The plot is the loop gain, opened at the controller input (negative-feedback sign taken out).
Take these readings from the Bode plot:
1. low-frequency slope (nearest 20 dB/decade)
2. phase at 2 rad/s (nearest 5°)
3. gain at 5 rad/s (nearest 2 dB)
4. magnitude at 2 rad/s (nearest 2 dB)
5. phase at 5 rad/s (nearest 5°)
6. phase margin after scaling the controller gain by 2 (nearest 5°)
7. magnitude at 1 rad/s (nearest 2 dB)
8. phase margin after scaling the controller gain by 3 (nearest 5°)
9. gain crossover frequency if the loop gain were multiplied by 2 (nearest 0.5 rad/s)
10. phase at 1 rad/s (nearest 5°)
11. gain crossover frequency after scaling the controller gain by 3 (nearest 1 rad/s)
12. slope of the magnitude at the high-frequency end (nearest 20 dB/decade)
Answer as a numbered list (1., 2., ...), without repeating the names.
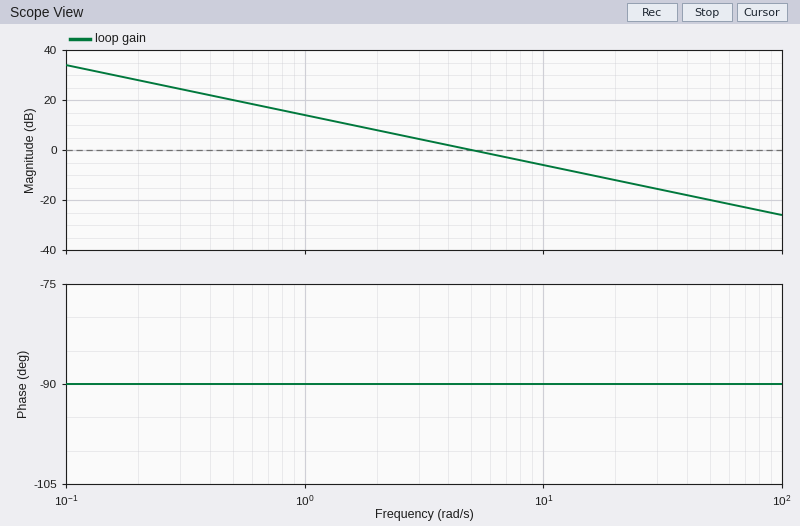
1. -20 dB/decade
2. -90°
3. 0 dB
4. 8 dB
5. -90°
6. 90°
7. 14 dB
8. 90°
9. 10.0 rad/s
10. -90°
11. 15 rad/s
12. -20 dB/decade
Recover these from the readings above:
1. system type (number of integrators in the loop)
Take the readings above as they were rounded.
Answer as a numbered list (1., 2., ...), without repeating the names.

1. 1
